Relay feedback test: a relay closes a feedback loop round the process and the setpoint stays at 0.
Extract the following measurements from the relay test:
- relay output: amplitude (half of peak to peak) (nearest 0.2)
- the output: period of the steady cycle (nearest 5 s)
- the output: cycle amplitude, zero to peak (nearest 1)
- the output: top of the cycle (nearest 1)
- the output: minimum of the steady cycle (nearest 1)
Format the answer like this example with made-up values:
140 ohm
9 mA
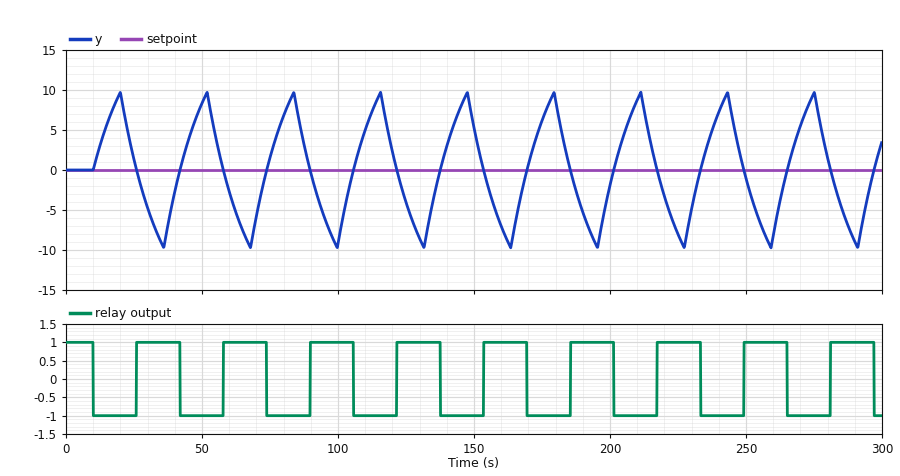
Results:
1.0
30 s
10
10
-10
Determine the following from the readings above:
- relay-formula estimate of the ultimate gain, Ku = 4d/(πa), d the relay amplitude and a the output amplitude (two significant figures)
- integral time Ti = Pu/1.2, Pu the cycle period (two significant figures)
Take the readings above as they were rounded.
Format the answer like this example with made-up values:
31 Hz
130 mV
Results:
0.13
25 s
